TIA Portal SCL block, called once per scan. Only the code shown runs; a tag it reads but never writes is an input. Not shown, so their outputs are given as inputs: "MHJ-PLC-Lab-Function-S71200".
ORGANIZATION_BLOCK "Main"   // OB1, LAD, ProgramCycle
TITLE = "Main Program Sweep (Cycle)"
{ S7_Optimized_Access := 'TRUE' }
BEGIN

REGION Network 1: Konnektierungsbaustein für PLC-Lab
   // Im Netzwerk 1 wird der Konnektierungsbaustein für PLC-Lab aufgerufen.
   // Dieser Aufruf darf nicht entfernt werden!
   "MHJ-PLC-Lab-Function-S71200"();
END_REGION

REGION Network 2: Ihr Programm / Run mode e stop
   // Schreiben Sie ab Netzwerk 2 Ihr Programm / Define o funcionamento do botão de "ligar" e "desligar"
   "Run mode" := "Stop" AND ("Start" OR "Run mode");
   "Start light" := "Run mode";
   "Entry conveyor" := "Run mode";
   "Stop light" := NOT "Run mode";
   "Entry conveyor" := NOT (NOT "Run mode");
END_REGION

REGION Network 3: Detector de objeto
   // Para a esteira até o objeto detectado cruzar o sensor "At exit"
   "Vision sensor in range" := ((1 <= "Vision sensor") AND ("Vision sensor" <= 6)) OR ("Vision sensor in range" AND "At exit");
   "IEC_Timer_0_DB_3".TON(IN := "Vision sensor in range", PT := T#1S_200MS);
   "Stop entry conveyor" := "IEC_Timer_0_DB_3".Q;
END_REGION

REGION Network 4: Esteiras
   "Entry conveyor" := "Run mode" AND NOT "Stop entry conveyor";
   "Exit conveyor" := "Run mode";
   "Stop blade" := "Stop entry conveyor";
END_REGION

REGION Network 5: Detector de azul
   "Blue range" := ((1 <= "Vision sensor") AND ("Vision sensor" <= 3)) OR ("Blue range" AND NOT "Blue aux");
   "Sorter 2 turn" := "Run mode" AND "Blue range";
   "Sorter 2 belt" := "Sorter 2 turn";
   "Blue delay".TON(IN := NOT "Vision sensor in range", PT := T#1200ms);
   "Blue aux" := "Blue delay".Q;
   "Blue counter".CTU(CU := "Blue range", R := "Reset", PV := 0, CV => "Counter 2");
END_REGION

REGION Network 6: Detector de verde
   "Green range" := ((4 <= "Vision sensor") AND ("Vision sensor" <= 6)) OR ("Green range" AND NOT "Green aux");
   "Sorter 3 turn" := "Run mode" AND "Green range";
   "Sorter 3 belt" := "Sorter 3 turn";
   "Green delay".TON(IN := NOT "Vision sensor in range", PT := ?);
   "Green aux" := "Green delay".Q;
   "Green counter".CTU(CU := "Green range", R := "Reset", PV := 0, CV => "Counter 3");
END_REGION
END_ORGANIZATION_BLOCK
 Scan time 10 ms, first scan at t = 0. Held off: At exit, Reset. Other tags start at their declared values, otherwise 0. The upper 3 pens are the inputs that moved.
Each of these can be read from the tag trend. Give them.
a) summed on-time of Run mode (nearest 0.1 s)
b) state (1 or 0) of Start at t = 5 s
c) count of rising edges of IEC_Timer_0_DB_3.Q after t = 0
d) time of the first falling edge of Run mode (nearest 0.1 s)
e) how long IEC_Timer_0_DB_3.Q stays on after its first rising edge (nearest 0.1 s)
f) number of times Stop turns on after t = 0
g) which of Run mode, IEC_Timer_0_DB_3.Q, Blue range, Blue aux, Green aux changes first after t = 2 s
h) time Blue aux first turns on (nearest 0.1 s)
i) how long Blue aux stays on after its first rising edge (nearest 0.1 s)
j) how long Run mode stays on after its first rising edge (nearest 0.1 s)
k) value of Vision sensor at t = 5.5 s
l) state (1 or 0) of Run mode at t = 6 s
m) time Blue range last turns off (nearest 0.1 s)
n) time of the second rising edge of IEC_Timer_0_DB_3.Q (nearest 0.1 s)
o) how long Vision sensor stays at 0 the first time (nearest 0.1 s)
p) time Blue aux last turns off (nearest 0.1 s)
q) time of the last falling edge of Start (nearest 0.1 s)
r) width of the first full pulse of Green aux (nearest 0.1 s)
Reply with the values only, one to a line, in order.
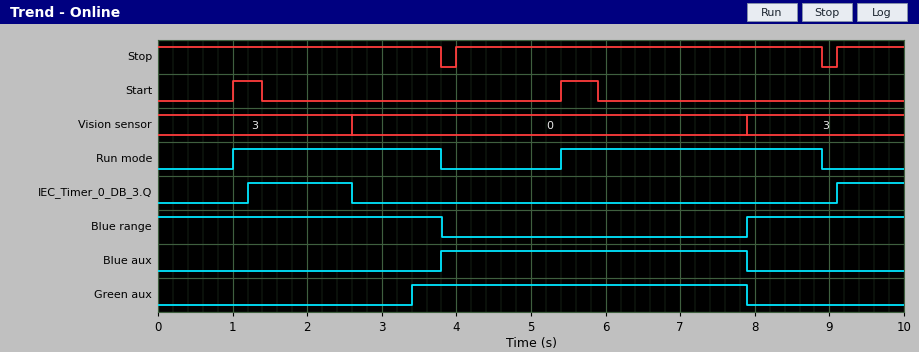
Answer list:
6.3 s
0
2
3.8 s
1.4 s
2
IEC_Timer_0_DB_3.Q
3.8 s
4.1 s
2.8 s
0
1
3.8 s
9.1 s
5.3 s
7.9 s
5.9 s
4.5 s
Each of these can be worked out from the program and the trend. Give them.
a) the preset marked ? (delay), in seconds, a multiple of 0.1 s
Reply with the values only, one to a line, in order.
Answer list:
0.8 s
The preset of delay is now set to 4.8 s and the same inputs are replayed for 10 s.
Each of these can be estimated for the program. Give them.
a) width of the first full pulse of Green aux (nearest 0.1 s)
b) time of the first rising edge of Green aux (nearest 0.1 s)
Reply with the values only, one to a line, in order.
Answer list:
0.5 s
7.4 s
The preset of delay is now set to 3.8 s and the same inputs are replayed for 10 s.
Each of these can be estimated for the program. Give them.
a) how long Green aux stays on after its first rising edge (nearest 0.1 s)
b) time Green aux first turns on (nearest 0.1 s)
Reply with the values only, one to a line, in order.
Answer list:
1.5 s
6.4 s
